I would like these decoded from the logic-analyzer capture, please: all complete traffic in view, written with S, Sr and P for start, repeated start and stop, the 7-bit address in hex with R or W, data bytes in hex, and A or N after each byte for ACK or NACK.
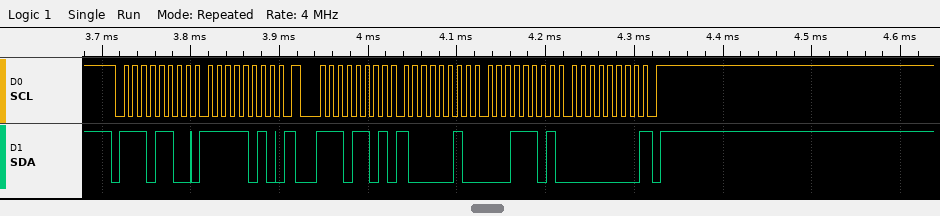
S 76W A FA A Sr 76R A 82 A 1D A 00 N P
